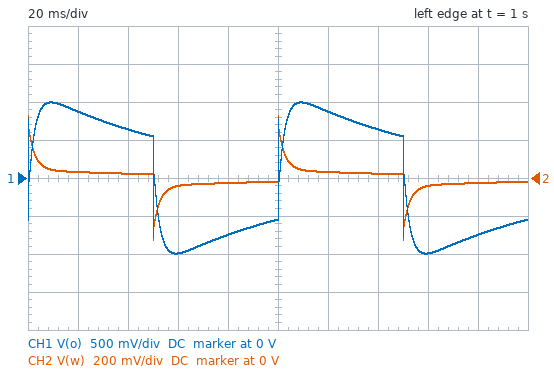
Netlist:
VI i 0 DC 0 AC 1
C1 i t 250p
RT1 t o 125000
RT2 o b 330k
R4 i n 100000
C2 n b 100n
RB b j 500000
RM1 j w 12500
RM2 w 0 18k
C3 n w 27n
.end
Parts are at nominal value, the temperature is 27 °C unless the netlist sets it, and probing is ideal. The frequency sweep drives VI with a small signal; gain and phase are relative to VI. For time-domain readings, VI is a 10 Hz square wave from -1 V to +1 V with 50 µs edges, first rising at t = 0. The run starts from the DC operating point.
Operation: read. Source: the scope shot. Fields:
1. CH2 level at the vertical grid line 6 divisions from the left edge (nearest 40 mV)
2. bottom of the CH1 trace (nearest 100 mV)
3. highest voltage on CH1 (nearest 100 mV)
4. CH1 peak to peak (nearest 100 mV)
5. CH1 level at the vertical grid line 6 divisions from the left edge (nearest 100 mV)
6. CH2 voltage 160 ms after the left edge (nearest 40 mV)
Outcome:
40 mV
-1.0 V
1.0 V
2.0 V
900 mV
-40 mV
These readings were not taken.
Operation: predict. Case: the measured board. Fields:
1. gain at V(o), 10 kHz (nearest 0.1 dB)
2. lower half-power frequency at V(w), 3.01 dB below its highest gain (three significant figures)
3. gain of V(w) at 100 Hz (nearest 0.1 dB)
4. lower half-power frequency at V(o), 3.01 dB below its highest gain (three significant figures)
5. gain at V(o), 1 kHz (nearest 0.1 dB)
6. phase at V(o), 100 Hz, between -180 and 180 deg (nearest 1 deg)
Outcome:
-2.3 dB
91.4 Hz
-17.7 dB
2.31 Hz
-7.0 dB
-37 deg
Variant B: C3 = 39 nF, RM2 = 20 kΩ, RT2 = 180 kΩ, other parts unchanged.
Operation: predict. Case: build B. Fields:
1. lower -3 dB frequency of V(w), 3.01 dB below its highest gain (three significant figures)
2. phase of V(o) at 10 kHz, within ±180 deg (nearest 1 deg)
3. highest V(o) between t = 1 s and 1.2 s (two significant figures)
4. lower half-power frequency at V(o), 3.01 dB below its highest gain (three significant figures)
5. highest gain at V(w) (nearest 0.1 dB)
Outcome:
81.0 Hz
8 deg
950 mV
2.23 Hz
-13.6 dB
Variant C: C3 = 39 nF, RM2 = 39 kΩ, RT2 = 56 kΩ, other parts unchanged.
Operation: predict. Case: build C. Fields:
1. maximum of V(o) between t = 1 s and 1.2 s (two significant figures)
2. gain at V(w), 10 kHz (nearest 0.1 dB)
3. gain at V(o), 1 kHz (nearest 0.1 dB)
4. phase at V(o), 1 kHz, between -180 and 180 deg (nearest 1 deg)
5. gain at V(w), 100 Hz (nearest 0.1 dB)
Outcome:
940 mV
-8.6 dB
-10.0 dB
12 deg
-11.6 dB
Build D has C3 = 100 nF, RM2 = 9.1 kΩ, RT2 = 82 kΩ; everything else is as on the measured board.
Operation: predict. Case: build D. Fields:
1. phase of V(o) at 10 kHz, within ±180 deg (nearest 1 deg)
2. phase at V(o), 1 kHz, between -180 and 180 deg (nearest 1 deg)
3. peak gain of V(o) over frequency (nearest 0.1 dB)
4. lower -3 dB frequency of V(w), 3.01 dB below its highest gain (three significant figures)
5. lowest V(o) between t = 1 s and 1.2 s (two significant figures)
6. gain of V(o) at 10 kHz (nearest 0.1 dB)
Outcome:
13 deg
39 deg
-2.8 dB
438 Hz
-780 mV
-7.0 dB
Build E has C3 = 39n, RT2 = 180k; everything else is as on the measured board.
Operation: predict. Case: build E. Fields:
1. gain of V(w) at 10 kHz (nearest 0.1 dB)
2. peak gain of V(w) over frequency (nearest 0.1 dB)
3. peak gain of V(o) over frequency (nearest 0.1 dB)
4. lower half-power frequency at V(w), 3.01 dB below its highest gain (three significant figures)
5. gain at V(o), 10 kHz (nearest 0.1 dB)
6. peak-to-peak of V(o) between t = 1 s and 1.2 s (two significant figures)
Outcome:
-14.4 dB
-14.3 dB
-2.0 dB
84.1 Hz
-3.7 dB
1.9 V
